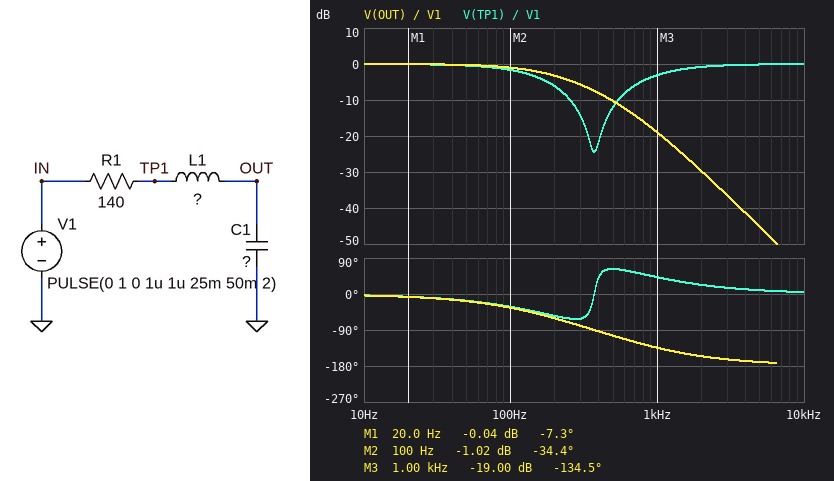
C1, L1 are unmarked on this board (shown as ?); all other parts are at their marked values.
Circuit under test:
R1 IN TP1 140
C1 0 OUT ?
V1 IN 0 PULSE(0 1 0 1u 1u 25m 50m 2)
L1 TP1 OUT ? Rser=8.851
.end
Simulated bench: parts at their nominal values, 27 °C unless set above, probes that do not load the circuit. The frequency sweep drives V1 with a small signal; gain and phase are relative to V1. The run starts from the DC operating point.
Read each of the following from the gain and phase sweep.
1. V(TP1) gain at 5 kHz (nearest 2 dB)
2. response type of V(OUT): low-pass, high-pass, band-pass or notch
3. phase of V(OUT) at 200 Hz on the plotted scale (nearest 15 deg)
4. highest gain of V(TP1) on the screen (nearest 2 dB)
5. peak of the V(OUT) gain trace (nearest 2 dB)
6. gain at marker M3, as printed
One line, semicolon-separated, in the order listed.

0 dB; low-pass; -60 deg; 0 dB; 0 dB; -19.00 dB
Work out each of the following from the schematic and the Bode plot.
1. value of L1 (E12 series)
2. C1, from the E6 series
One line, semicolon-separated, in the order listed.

27 mH; 6.8 µF
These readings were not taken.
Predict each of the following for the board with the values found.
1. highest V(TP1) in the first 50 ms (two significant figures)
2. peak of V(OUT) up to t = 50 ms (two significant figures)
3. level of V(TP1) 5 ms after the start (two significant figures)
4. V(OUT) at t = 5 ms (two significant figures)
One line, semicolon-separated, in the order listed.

1.0 V; 1.0 V; 1.0 V; 1.0 V
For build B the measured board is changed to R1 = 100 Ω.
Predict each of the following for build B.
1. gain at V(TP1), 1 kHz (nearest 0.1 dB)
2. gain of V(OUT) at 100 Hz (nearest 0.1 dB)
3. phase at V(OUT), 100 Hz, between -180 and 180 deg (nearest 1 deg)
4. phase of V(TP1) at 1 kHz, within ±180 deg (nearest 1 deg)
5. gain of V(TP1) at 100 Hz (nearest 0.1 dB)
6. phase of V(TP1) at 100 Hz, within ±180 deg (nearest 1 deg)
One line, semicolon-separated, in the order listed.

-1.9 dB; -0.3 dB; -27 deg; 33 deg; -1.0 dB; -24 deg
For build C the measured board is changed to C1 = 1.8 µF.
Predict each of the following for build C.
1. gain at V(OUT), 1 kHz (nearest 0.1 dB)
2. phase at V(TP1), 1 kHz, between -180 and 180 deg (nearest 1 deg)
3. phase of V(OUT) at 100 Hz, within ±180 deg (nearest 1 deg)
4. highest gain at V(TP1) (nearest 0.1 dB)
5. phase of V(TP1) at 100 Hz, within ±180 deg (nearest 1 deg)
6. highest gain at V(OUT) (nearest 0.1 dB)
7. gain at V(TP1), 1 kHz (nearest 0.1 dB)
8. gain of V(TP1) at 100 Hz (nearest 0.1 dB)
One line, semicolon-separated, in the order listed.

-5.7 dB; 55 deg; -10 deg; 0 dB; -9 deg; 0.3 dB; -6.3 dB; -0.1 dB
